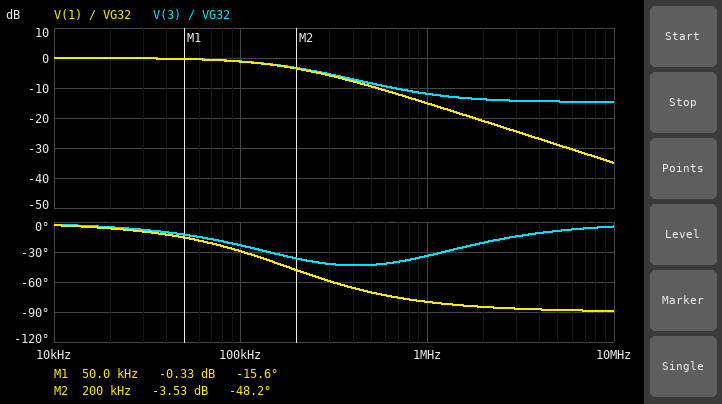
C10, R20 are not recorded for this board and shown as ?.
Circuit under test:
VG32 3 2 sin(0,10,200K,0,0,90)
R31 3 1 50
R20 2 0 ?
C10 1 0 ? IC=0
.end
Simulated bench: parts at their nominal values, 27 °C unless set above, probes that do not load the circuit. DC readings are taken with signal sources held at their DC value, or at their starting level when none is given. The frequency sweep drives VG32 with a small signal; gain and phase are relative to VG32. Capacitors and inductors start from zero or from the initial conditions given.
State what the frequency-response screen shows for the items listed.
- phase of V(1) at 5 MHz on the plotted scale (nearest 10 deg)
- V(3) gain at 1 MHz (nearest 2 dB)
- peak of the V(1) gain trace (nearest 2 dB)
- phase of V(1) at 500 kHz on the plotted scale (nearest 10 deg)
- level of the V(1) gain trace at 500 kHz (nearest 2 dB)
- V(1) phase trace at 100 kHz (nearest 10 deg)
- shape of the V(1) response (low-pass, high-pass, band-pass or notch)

-90 deg
-12 dB
0 dB
-70 deg
-10 dB
-30 deg
low-pass
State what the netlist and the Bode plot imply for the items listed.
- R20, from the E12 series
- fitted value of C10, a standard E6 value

220 Ω
3.3 nF
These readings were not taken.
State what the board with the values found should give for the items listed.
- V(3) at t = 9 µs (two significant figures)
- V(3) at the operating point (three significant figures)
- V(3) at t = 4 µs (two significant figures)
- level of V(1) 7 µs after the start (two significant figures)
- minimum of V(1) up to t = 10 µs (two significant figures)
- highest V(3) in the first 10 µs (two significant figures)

-2.2 V
10.0 V
-2.2 V
-670 mV
-6.8 V
6.8 V
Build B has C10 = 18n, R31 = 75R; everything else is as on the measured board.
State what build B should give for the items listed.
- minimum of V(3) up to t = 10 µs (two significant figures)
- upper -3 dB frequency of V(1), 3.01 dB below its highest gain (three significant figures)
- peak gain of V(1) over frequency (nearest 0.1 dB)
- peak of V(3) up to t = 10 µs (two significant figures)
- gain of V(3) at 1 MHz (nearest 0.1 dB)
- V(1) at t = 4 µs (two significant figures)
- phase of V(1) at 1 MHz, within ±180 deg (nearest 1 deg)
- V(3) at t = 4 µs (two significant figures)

-3.0 V
30.0 kHz
0 dB
2.9 V
-11.8 dB
-1.4 V
-88 deg
-280 mV
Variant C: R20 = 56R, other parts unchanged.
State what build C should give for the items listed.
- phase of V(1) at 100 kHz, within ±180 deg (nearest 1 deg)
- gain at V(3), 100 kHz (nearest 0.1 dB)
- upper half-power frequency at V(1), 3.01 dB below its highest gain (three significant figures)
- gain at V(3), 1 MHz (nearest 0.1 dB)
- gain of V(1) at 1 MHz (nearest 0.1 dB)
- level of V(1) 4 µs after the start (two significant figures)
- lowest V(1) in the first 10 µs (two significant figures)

-12 deg
-0.2 dB
455 kHz
-4.5 dB
-7.7 dB
-910 mV
-9.2 V
